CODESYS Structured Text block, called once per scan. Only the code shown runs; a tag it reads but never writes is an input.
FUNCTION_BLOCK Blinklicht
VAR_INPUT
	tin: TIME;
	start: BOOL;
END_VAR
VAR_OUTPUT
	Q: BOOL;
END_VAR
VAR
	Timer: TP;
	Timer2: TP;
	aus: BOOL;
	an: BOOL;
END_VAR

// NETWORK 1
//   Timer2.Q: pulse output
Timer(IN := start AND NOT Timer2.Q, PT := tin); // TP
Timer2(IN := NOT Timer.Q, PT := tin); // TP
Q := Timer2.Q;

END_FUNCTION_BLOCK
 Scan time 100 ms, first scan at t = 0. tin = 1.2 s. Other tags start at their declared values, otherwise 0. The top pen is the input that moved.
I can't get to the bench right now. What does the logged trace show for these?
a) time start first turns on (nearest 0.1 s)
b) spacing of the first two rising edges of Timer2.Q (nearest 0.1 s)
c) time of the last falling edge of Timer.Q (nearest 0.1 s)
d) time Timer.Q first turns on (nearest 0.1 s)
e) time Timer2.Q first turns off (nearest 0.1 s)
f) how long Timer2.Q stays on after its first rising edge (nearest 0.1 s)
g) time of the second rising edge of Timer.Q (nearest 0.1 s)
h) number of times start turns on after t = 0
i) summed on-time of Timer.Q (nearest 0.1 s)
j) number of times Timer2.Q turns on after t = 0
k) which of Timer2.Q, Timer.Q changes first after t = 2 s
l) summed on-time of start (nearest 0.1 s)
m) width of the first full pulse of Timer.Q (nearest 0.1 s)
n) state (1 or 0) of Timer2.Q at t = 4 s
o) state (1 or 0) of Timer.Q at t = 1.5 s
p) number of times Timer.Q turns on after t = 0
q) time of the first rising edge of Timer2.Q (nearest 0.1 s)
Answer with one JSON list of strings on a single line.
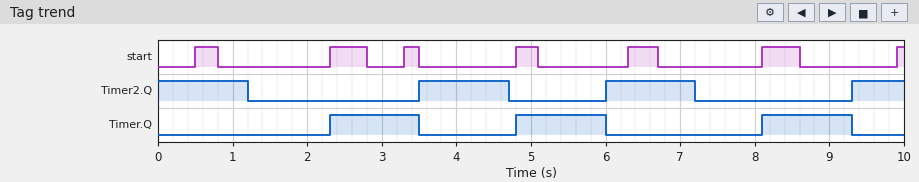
["0.5 s", "2.5 s", "9.3 s", "2.3 s", "1.2 s", "1.2 s", "4.8 s", "7", "3.6 s", "3", "Timer.Q", "2.3 s", "1.2 s", "1", "0", "3", "3.5 s"]
